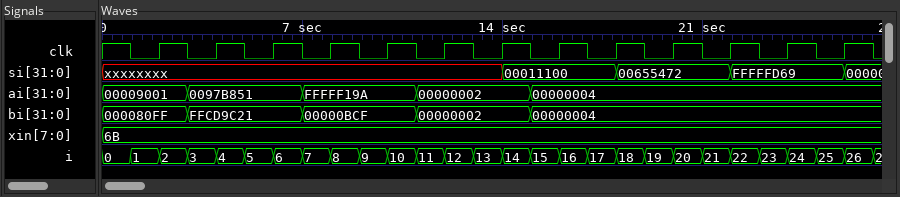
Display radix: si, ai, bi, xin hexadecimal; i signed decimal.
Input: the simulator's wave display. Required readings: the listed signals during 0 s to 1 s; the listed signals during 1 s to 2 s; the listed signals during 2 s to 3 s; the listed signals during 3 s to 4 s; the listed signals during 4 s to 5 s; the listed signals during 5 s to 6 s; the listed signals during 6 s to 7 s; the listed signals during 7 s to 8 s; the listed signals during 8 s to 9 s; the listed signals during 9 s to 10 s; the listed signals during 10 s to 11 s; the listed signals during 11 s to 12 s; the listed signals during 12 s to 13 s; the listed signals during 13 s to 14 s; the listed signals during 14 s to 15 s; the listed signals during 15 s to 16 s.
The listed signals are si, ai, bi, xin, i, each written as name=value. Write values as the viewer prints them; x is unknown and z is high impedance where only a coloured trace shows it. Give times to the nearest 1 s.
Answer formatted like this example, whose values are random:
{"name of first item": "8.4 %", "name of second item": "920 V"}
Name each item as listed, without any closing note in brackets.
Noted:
{"the listed signals during 0 s to 1 s": "si=xxxxxxxx, ai=00009001, bi=000080FF, xin=6B, i=0", "the listed signals during 1 s to 2 s": "si=xxxxxxxx, ai=00009001, bi=000080FF, xin=6B, i=1", "the listed signals during 2 s to 3 s": "si=xxxxxxxx, ai=00009001, bi=000080FF, xin=6B, i=2", "the listed signals during 3 s to 4 s": "si=xxxxxxxx, ai=0097B851, bi=FFCD9C21, xin=6B, i=3", "the listed signals during 4 s to 5 s": "si=xxxxxxxx, ai=0097B851, bi=FFCD9C21, xin=6B, i=4", "the listed signals during 5 s to 6 s": "si=xxxxxxxx, ai=0097B851, bi=FFCD9C21, xin=6B, i=5", "the listed signals during 6 s to 7 s": "si=xxxxxxxx, ai=0097B851, bi=FFCD9C21, xin=6B, i=6", "the listed signals during 7 s to 8 s": "si=xxxxxxxx, ai=FFFFF19A, bi=00000BCF, xin=6B, i=7", "the listed signals during 8 s to 9 s": "si=xxxxxxxx, ai=FFFFF19A, bi=00000BCF, xin=6B, i=8", "the listed signals during 9 s to 10 s": "si=xxxxxxxx, ai=FFFFF19A, bi=00000BCF, xin=6B, i=9", "the listed signals during 10 s to 11 s": "si=xxxxxxxx, ai=FFFFF19A, bi=00000BCF, xin=6B, i=10", "the listed signals during 11 s to 12 s": "si=xxxxxxxx, ai=00000002, bi=00000002, xin=6B, i=11", "the listed signals during 12 s to 13 s": "si=xxxxxxxx, ai=00000002, bi=00000002, xin=6B, i=12", "the listed signals during 13 s to 14 s": "si=xxxxxxxx, ai=00000002, bi=00000002, xin=6B, i=13", "the listed signals during 14 s to 15 s": "si=00011100, ai=00000002, bi=00000002, xin=6B, i=14", "the listed signals during 15 s to 16 s": "si=00011100, ai=00000004, bi=00000004, xin=6B, i=15"}
